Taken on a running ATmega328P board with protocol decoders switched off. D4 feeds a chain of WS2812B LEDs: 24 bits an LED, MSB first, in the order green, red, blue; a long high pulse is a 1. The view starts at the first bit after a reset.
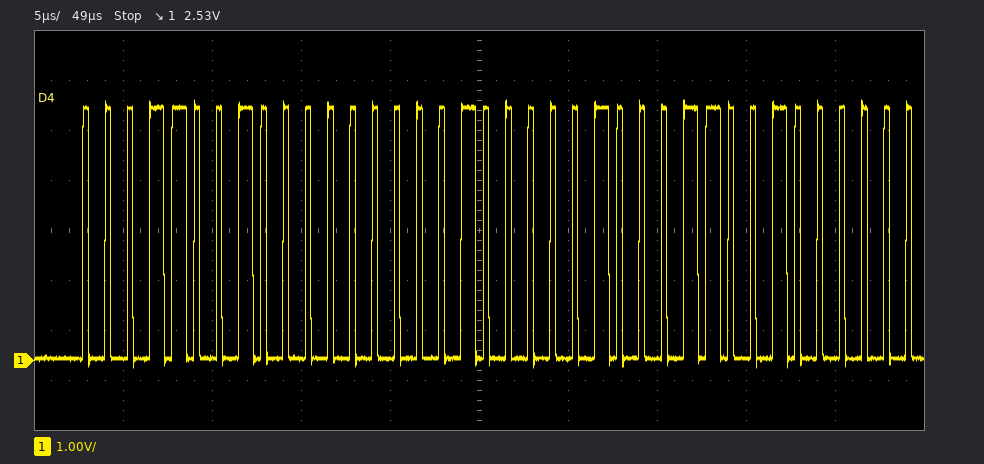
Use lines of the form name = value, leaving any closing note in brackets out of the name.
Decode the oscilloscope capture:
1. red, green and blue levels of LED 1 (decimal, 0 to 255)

red, green and blue levels of LED 1 = 0, 25, 65
